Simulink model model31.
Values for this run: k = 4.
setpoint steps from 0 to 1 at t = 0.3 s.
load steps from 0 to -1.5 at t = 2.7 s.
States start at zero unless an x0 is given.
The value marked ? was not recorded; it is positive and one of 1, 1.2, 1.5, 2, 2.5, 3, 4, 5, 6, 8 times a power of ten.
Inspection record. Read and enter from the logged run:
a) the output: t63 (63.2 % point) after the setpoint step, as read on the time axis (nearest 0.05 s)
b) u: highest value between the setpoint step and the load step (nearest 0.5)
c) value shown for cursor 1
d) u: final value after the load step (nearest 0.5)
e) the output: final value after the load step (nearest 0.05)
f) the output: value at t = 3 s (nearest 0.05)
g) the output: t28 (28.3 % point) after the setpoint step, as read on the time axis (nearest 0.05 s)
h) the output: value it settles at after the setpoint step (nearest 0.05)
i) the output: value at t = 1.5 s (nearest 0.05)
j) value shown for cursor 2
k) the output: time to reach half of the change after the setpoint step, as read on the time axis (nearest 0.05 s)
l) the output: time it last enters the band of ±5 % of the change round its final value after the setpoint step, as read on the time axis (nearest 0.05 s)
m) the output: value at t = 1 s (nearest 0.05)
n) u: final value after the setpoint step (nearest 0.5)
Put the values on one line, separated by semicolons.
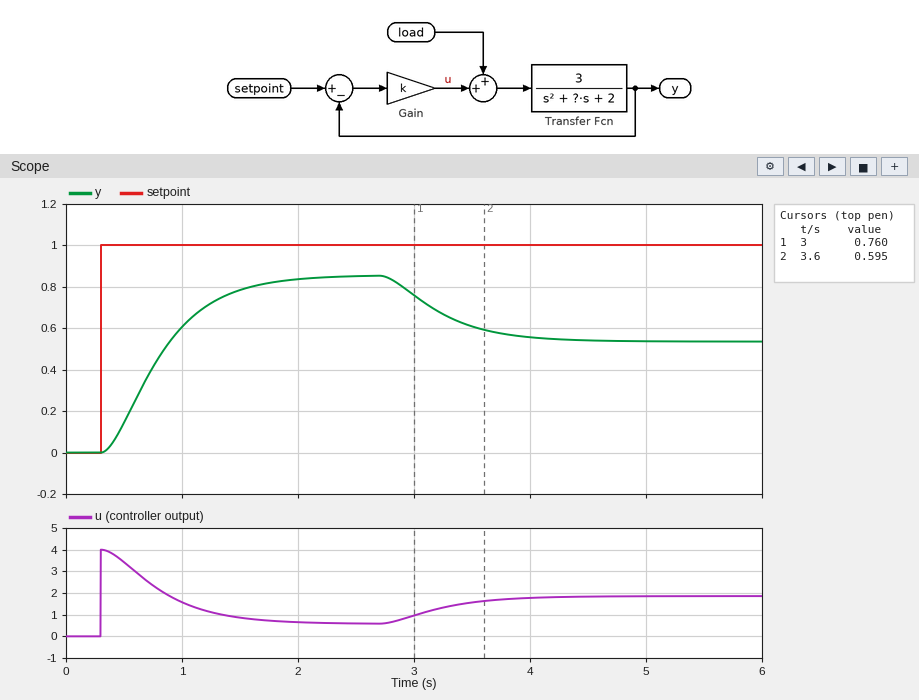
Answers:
0.90 s; 4.0; 0.760; 2.0; 0.55; 0.75; 0.60 s; 0.85; 0.80; 0.595; 0.75 s; 1.70 s; 0.60; 0.5
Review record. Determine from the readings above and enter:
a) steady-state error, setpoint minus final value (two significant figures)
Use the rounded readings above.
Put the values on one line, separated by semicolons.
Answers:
0.15
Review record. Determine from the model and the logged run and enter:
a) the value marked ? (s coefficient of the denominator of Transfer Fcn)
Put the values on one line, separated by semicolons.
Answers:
8
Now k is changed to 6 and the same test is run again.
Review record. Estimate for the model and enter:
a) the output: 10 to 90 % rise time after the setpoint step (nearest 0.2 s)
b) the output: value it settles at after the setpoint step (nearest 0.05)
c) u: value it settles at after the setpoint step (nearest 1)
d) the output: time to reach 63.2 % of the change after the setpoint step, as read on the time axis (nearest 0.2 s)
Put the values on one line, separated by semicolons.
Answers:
0.6 s; 0.90; 1; 0.8 s
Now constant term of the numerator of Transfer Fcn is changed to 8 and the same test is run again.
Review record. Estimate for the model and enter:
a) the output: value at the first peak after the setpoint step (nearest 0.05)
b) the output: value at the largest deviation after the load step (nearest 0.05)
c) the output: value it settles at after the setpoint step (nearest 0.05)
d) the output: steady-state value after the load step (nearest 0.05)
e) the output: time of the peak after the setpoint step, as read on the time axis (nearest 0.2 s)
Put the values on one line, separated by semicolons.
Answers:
1.00; 0.55; 0.95; 0.60; 1.0 s
